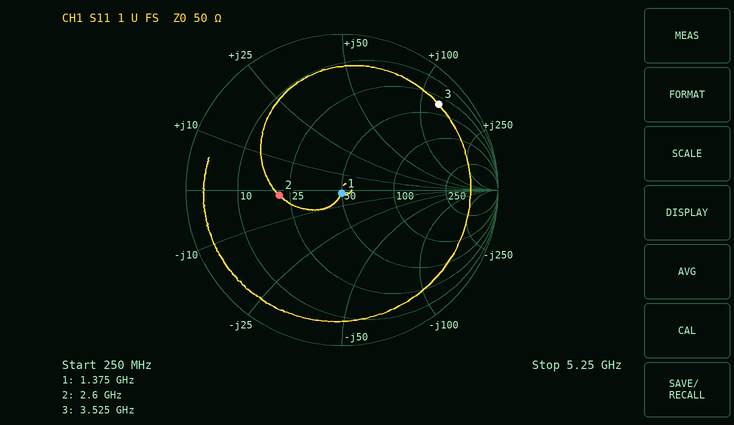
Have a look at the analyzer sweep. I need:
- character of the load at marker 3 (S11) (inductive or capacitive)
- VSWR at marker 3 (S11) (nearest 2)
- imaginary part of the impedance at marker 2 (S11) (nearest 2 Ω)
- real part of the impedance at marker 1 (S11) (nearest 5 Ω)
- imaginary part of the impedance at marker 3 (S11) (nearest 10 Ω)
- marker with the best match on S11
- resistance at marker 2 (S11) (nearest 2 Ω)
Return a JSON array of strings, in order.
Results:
["inductive", "10", "-2 Ω", "50 Ω", "+120 Ω", "marker 1", "22 Ω"]
